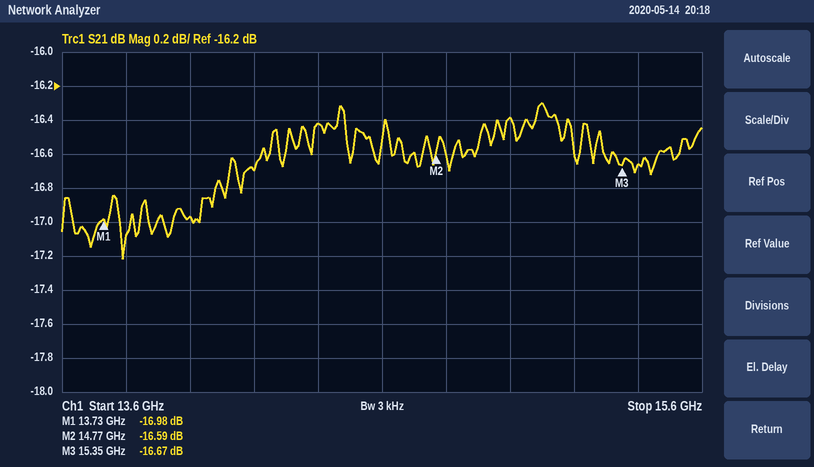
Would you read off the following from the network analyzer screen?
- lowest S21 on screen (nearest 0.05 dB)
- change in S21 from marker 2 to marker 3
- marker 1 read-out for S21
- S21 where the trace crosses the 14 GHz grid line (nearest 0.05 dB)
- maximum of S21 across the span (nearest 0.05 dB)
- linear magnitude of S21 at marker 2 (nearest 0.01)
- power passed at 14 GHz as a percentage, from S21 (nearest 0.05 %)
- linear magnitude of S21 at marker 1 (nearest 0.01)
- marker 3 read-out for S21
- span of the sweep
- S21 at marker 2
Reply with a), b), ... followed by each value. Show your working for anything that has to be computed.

a) -17.20 dB
b) -16.67 − (-16.59) = -0.08 dB
c) -16.98 dB
d) -16.95 dB
e) -16.30 dB
f) 10^(-16.59/20) ≈ 0.15
g) 10^(-16.95/10) ≈ 2.02 %, so 2.00 % to the nearest 0.05 %
h) 10^(-16.98/20) ≈ 0.14
i) -16.67 dB
j) 2 GHz
k) -16.59 dB
